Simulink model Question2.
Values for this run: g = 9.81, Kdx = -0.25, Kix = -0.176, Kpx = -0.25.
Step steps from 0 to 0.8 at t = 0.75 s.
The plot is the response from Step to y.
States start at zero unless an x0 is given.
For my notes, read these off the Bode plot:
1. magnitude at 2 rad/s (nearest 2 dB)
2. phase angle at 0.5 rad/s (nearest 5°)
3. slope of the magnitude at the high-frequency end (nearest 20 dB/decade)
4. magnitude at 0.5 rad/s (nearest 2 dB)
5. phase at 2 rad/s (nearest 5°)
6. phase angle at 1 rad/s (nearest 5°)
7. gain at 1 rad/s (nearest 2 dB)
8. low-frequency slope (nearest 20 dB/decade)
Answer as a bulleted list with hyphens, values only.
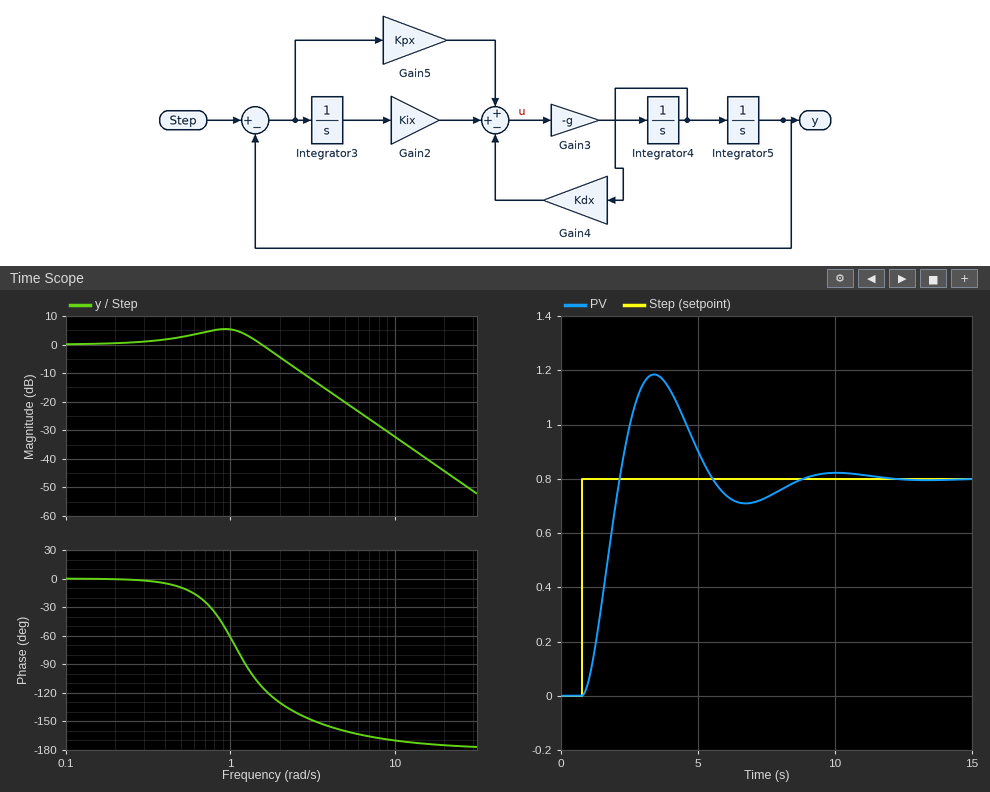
- -4 dB
- -10°
- -40 dB/decade
- 2 dB
- -130°
- -60°
- 6 dB
- 0 dB/decade
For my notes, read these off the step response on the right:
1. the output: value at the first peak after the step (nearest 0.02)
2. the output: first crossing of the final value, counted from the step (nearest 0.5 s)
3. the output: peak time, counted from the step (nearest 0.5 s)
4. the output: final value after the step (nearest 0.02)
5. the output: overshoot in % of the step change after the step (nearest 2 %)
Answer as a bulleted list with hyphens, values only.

- 1.18
- 1.5 s
- 2.5 s
- 0.80
- 48 %
